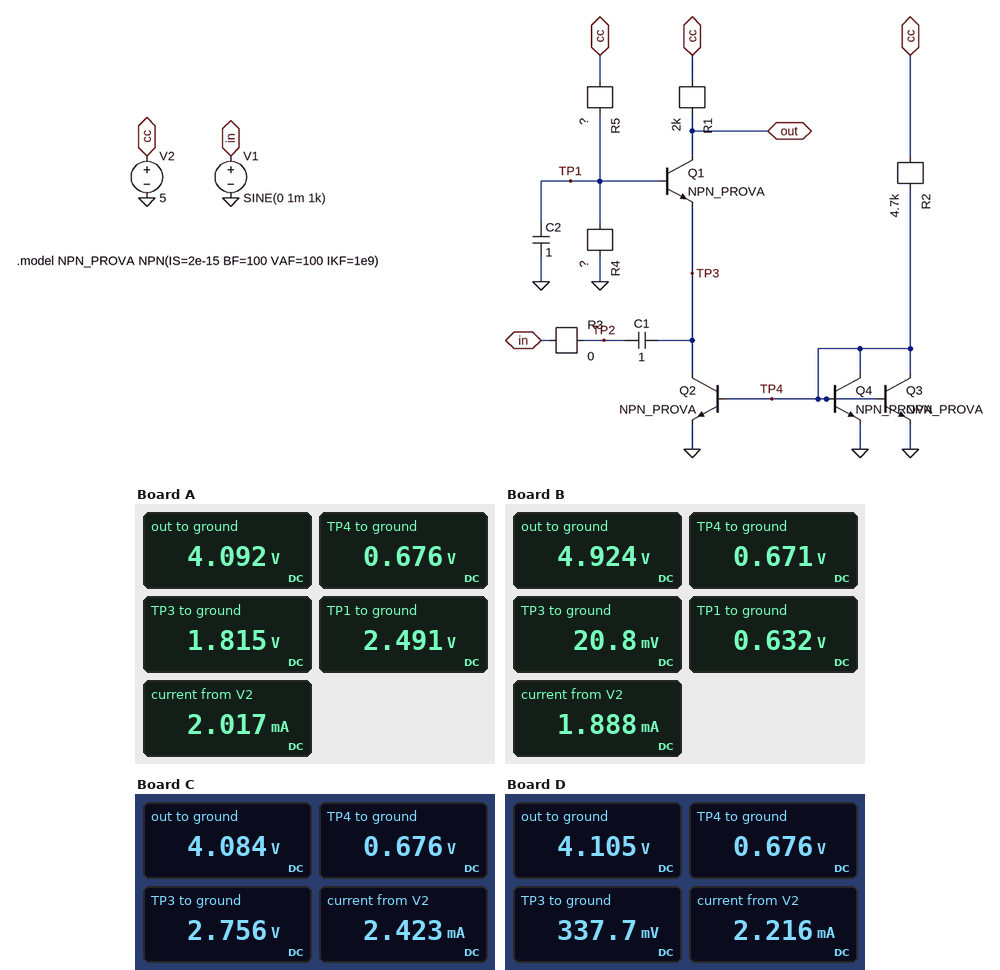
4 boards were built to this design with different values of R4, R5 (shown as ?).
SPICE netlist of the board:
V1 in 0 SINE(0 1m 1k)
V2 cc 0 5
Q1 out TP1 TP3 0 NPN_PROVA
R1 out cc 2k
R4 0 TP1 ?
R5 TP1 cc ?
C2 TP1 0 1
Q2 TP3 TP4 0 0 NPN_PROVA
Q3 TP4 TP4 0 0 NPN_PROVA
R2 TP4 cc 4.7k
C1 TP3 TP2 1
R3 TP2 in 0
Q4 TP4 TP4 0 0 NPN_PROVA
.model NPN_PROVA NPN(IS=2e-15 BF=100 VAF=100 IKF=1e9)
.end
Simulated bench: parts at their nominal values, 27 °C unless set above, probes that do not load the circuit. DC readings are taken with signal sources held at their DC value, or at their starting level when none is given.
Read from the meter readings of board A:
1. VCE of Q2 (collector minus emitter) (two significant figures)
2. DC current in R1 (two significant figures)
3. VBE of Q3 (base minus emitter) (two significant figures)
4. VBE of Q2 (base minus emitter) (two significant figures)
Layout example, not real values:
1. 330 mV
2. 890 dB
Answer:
1. 1.8 V
2. 450 µA
3. 680 mV
4. 680 mV
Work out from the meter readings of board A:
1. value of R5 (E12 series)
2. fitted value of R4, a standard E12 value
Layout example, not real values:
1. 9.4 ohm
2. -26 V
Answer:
1. 3.9 kΩ
2. 3.9 kΩ
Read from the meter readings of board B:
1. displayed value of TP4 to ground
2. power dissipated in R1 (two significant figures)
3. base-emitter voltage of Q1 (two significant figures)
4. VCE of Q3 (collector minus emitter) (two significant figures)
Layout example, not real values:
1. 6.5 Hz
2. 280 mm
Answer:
1. 0.671 V
2. 2.9 µW
3. 610 mV
4. 670 mV
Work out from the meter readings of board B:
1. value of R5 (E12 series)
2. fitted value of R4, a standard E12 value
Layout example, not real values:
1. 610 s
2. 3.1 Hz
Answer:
1. 4.7 kΩ
2. 680 Ω
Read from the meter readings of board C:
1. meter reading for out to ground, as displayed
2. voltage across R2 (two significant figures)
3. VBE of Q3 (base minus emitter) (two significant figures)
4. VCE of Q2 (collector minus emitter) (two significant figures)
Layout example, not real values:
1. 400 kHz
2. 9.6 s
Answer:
1. 4.084 V
2. 4.3 V
3. 680 mV
4. 2.8 V
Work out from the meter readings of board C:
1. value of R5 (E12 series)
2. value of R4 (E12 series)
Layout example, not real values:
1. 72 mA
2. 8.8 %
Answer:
1. 1.5 kΩ
2. 3.3 kΩ
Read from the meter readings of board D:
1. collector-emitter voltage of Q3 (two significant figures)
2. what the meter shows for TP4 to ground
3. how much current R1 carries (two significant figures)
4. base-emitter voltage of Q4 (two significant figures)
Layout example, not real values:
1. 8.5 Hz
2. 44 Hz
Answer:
1. 680 mV
2. 0.676 V
3. 450 µA
4. 680 mV
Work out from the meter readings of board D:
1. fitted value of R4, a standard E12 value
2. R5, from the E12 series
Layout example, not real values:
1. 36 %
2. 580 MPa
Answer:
1. 1.2 kΩ
2. 4.7 kΩ
